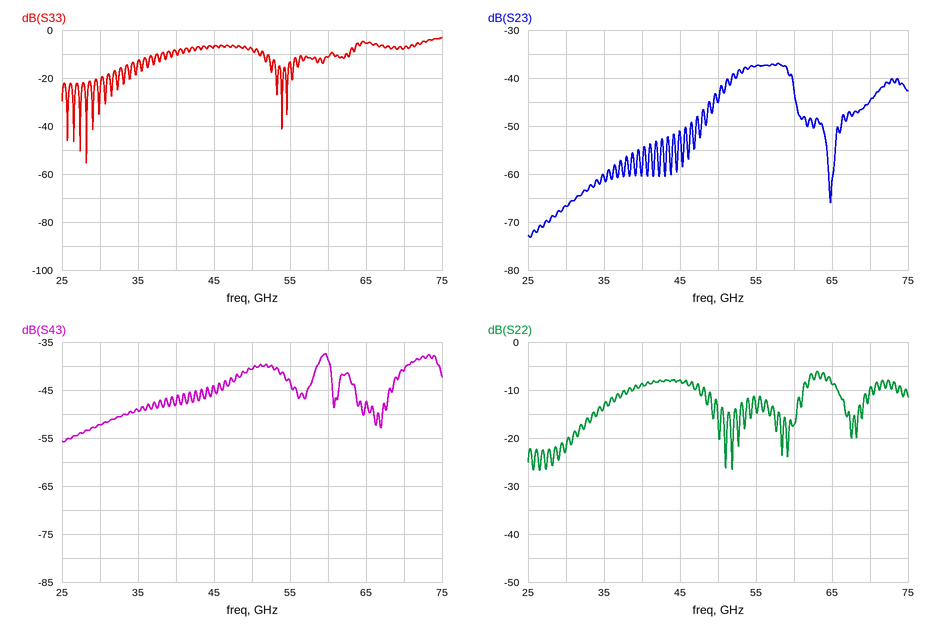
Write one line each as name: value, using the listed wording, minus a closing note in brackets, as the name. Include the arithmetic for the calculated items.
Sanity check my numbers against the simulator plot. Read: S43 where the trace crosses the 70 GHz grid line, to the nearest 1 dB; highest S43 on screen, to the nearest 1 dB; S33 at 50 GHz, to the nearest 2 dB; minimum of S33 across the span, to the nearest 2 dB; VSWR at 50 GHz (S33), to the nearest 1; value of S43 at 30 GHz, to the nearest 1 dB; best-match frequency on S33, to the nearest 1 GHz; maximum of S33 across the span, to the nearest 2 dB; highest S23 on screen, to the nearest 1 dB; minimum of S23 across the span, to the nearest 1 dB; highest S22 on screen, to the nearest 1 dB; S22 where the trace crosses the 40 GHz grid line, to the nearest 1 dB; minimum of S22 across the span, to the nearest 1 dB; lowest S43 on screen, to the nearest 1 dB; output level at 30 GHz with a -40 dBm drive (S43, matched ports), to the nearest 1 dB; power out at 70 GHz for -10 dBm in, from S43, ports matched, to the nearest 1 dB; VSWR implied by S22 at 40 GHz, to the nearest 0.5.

S43 where the trace crosses the 70 GHz grid line, to the nearest 1 dB: -41 dB
highest S43 on screen, to the nearest 1 dB: -37 dB
S33 at 50 GHz, to the nearest 2 dB: -8 dB
minimum of S33 across the span, to the nearest 2 dB: -56 dB
VSWR at 50 GHz (S33), to the nearest 1: |Γ| = 10^(-8/20) = 0.3981; VSWR = (1 + 0.3981)/(1 − 0.3981) ≈ 2
value of S43 at 30 GHz, to the nearest 1 dB: -52 dB
best-match frequency on S33, to the nearest 1 GHz: 28 GHz
maximum of S33 across the span, to the nearest 2 dB: -4 dB
highest S23 on screen, to the nearest 1 dB: -37 dB
minimum of S23 across the span, to the nearest 1 dB: -73 dB
highest S22 on screen, to the nearest 1 dB: -6 dB
S22 where the trace crosses the 40 GHz grid line, to the nearest 1 dB: -9 dB
minimum of S22 across the span, to the nearest 1 dB: -27 dB
lowest S43 on screen, to the nearest 1 dB: -56 dB
output level at 30 GHz with a -40 dBm drive (S43, matched ports), to the nearest 1 dB: -40 dBm + (-52 dB) = -92 dBm
power out at 70 GHz for -10 dBm in, from S43, ports matched, to the nearest 1 dB: -10 dBm + (-41 dB) = -51 dBm
VSWR implied by S22 at 40 GHz, to the nearest 0.5: |Γ| = 10^(-9/20) = 0.3548; VSWR = (1 + 0.3548)/(1 − 0.3548) ≈ 2.10, so 2.0 to the nearest 0.5
